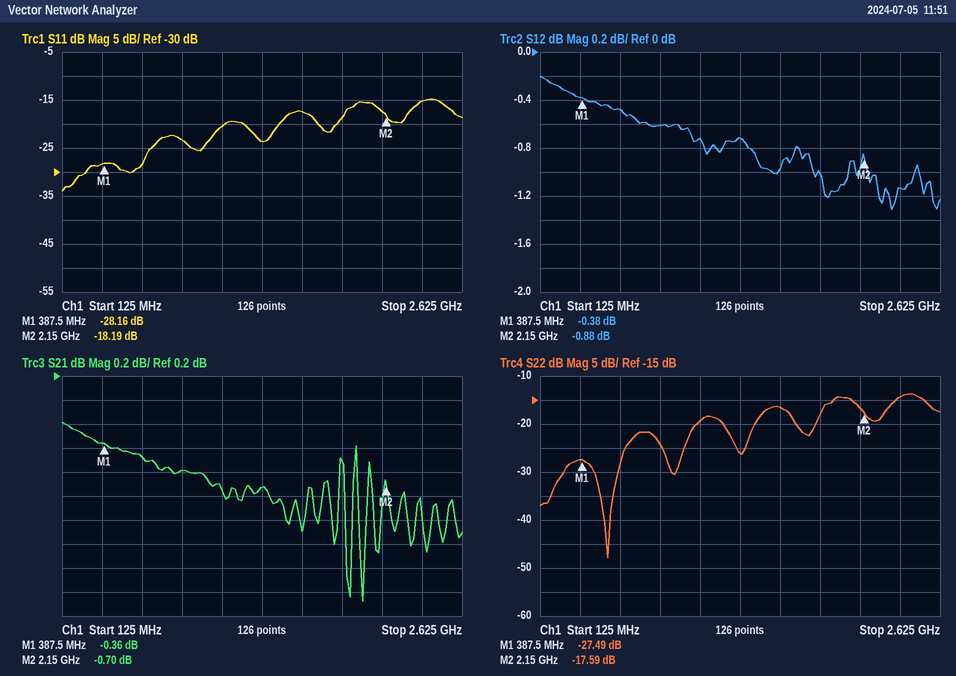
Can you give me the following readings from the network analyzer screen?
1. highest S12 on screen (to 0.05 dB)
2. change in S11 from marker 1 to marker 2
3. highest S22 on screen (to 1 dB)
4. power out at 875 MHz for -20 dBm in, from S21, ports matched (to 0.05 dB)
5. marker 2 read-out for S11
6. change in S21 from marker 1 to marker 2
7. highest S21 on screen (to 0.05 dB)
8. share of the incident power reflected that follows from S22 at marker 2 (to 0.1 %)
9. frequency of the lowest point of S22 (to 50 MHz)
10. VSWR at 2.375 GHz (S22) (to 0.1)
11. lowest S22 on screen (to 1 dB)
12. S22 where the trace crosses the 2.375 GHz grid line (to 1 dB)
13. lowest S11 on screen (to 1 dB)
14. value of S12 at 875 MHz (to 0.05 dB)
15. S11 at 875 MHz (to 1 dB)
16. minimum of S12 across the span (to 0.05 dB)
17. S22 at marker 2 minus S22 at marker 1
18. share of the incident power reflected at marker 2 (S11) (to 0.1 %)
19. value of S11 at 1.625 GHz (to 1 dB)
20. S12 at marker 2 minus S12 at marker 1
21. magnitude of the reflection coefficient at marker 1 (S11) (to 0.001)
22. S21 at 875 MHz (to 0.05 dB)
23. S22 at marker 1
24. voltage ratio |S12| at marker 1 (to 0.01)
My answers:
-0.20 dB
9.97 dB
-14 dB
-20.60 dBm
-18.19 dB
-0.34 dB
-0.20 dB
1.7 %
550 MHz
1.5
-48 dB
-14 dB
-34 dB
-0.60 dB
-23 dB
-1.30 dB
9.90 dB
1.5 %
-17 dB
-0.50 dB
0.039
-0.60 dB
-27.49 dB
0.96
